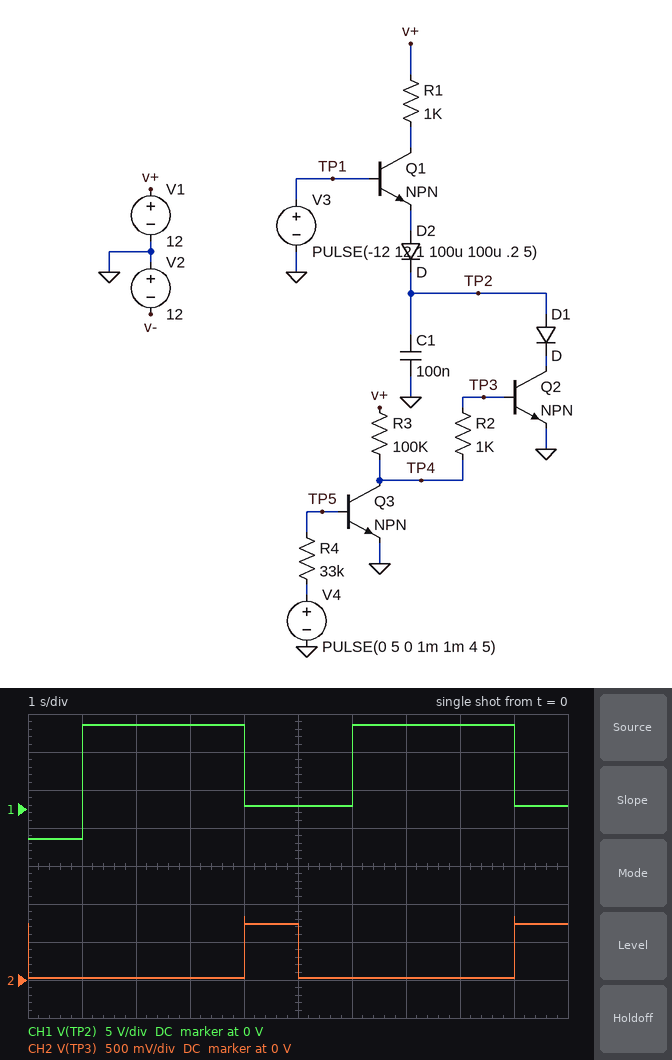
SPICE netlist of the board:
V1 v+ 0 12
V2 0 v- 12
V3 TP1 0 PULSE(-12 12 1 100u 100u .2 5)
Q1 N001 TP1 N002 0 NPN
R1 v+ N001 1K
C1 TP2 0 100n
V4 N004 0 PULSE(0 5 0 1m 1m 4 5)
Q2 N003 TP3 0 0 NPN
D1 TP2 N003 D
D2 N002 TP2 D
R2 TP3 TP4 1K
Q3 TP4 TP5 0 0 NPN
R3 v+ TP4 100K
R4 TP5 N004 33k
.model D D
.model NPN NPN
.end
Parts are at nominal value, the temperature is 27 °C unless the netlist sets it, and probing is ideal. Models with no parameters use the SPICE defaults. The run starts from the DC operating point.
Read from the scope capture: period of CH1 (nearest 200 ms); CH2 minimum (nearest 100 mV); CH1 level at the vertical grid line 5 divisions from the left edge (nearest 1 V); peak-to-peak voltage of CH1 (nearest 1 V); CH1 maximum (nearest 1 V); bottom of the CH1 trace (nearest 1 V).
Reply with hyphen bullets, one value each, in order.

- 5.0 s
- 0 V
- 0 V
- 15 V
- 11 V
- -4 V
